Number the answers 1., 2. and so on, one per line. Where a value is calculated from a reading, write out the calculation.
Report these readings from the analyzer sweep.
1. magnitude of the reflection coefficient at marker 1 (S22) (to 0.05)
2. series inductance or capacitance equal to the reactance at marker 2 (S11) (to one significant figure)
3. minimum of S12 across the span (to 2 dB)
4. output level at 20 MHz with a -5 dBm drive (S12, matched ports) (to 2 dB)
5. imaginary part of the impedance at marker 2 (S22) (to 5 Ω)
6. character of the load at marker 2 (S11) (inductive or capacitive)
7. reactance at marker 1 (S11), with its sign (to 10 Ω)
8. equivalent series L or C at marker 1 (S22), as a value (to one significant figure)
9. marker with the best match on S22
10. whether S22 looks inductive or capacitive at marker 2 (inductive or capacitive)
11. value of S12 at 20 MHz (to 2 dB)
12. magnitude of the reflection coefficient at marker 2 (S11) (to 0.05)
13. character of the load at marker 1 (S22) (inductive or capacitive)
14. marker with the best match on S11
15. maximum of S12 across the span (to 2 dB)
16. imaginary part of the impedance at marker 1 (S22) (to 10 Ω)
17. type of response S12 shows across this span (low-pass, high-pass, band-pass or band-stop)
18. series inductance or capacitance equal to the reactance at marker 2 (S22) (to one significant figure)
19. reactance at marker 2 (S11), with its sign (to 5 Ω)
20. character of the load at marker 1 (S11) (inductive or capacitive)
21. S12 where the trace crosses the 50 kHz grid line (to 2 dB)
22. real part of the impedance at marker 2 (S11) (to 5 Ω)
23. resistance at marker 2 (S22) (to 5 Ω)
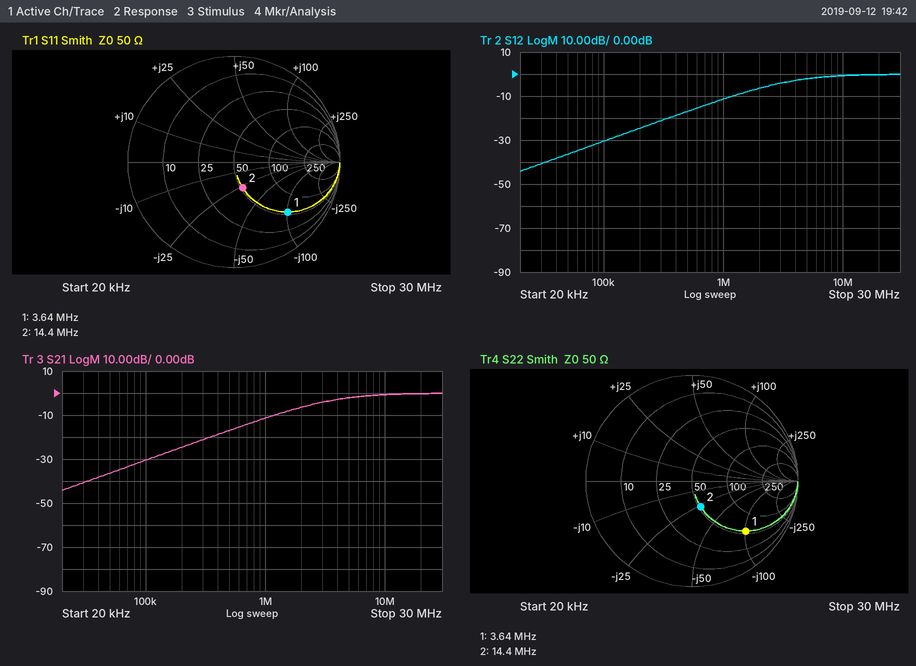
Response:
1. 0.70
2. C = 1/(2π × 14.4 MHz × 25 Ω) ≈ 442 pF, so 400 pF to one significant figure
3. -44 dB
4. -5 dBm + (0 dB) = -6 dBm
5. -25 Ω
6. capacitive
7. -100 Ω
8. C = 1/(2π × 3.64 MHz × 100 Ω) ≈ 437 pF, so 400 pF to one significant figure
9. marker 2
10. capacitive
11. 0 dB
12. 0.25
13. capacitive
14. marker 2
15. 0 dB
16. -100 Ω
17. high-pass
18. C = 1/(2π × 14.4 MHz × 25 Ω) ≈ 442 pF, so 400 pF to one significant figure
19. -25 Ω
20. capacitive
21. -36 dB
22. 50 Ω
23. 50 Ω
